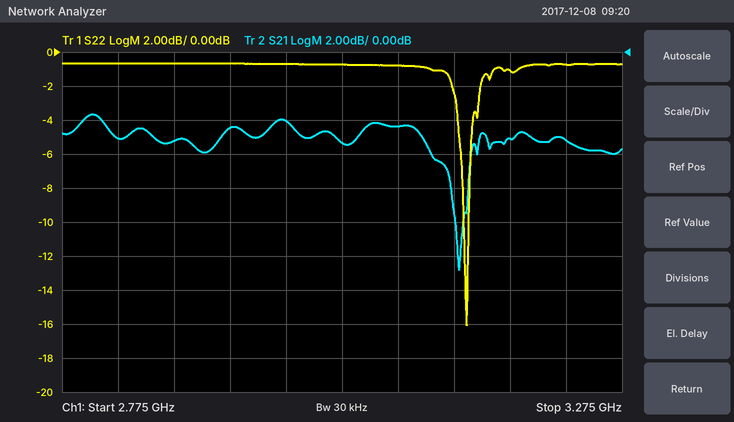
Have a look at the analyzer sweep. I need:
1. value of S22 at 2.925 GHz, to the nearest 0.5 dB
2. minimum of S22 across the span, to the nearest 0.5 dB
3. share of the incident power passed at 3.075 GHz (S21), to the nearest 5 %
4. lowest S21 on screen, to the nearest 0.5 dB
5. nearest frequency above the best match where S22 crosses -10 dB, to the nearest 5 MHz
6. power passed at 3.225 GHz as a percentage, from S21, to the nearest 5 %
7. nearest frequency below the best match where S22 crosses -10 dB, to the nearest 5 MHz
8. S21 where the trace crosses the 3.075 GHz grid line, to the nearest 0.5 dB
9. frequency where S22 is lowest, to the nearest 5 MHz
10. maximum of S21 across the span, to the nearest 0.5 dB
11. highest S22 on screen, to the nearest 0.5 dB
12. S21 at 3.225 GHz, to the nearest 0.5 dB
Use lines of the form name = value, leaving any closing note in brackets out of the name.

value of S22 at 2.925 GHz, to the nearest 0.5 dB = -0.5 dB
minimum of S22 across the span, to the nearest 0.5 dB = -16.0 dB
share of the incident power passed at 3.075 GHz (S21), to the nearest 5 % = 35 %
lowest S21 on screen, to the nearest 0.5 dB = -13.0 dB
nearest frequency above the best match where S22 crosses -10 dB, to the nearest 5 MHz = 3.140 GHz
power passed at 3.225 GHz as a percentage, from S21, to the nearest 5 % = 30 %
nearest frequency below the best match where S22 crosses -10 dB, to the nearest 5 MHz = 3.135 GHz
S21 where the trace crosses the 3.075 GHz grid line, to the nearest 0.5 dB = -4.5 dB
frequency where S22 is lowest, to the nearest 5 MHz = 3.135 GHz
maximum of S21 across the span, to the nearest 0.5 dB = -3.5 dB
highest S22 on screen, to the nearest 0.5 dB = -0.5 dB
S21 at 3.225 GHz, to the nearest 0.5 dB = -5.0 dB
